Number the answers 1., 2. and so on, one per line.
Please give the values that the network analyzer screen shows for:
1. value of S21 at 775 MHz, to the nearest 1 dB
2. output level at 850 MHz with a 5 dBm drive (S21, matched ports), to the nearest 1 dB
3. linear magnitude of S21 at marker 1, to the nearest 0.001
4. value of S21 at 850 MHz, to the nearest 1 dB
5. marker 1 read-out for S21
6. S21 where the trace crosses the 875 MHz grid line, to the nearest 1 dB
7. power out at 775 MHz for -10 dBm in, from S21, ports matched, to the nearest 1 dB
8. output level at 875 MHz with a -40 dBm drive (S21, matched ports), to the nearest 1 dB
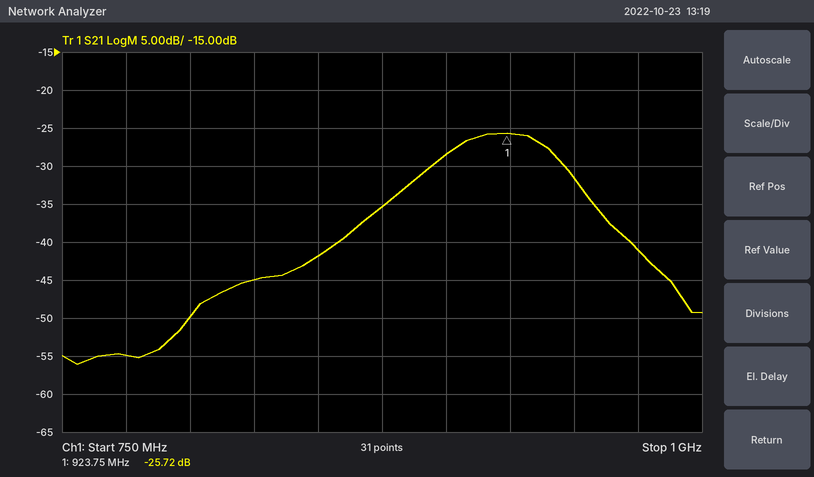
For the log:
1. -55 dB
2. -37 dBm
3. 0.052
4. -42 dB
5. -25.72 dB
6. -35 dB
7. -65 dBm
8. -75 dBm
